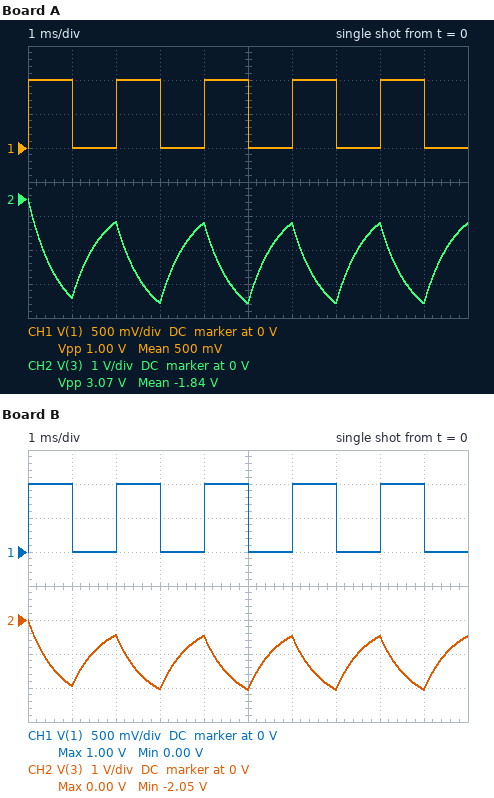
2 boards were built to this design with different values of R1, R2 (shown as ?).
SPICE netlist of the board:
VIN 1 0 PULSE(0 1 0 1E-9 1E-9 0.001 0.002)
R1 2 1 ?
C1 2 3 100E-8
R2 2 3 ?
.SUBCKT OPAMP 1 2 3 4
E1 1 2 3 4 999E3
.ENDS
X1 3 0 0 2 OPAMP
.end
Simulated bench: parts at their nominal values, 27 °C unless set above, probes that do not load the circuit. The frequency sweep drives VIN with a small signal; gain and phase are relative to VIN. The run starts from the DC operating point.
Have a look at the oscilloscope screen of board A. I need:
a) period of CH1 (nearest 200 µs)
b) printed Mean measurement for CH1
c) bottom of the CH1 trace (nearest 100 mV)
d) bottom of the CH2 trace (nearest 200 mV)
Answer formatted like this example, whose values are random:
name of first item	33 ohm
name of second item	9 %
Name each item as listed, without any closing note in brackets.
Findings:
period of CH1	2.0 ms
printed Mean measurement for CH1	500 mV
bottom of the CH1 trace	0 V
bottom of the CH2 trace	-3.0 V
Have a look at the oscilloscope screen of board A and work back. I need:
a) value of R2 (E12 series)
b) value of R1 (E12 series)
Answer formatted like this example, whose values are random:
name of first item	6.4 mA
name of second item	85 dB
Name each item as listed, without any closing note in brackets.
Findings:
value of R2	680 Ω
value of R1	180 Ω
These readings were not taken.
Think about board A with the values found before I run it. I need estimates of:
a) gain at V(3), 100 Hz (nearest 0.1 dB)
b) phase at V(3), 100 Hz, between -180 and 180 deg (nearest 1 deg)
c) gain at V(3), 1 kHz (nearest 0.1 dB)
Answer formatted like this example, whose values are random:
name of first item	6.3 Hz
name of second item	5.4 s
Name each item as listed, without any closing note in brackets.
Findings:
gain at V(3), 100 Hz	10.8 dB
phase at V(3), 100 Hz, between -180 and 180 deg	157 deg
gain at V(3), 1 kHz	-1.3 dB
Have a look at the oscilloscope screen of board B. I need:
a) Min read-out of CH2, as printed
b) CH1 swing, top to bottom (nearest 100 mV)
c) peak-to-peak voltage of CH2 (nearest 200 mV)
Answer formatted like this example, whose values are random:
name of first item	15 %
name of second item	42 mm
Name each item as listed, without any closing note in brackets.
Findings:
Min read-out of CH2, as printed	-2.05 V
CH1 swing, top to bottom	1.0 V
peak-to-peak voltage of CH2	2.0 V
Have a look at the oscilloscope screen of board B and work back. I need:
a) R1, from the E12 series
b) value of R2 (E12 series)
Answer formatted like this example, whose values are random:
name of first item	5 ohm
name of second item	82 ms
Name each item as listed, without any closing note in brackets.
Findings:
R1, from the E12 series	270 Ω
value of R2	680 Ω
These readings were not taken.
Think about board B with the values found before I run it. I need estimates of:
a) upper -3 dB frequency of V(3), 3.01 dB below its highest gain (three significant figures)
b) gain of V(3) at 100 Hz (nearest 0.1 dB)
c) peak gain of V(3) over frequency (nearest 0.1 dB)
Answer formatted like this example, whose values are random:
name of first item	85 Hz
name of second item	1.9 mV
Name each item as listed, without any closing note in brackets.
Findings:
upper -3 dB frequency of V(3), 3.01 dB below its highest gain	234 Hz
gain of V(3) at 100 Hz	7.3 dB
peak gain of V(3) over frequency	8.0 dB
